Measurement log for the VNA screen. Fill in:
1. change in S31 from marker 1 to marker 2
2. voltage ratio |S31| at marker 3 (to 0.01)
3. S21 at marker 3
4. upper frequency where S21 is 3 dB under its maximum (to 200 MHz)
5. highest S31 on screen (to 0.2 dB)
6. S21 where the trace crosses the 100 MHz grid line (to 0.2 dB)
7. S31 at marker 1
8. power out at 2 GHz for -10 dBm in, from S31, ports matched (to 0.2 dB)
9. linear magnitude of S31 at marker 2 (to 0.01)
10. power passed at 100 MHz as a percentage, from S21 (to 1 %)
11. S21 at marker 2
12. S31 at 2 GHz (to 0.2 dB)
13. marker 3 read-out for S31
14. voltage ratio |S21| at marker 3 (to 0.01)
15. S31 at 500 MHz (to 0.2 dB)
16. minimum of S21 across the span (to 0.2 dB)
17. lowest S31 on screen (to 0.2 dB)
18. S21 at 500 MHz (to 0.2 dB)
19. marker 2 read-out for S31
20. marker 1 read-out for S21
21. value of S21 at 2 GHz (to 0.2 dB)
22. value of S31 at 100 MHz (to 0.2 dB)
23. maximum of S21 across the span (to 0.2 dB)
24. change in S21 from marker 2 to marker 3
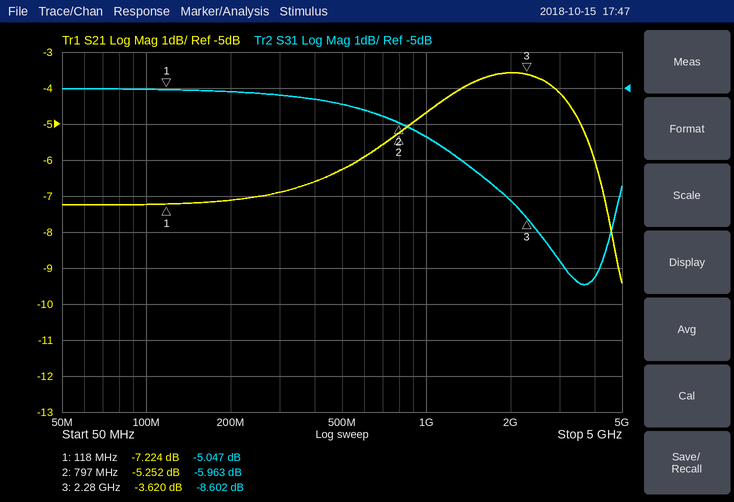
-0.916 dB
0.37
-3.620 dB
4.2 GHz
-5.0 dB
-7.2 dB
-5.047 dB
-18.2 dBm
0.50
19 %
-5.252 dB
-8.2 dB
-8.602 dB
0.66
-5.4 dB
-9.4 dB
-10.4 dB
-6.2 dB
-5.963 dB
-7.224 dB
-3.6 dB
-5.0 dB
-3.6 dB
1.632 dB
